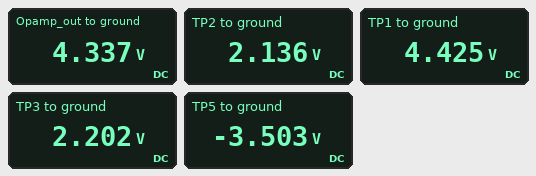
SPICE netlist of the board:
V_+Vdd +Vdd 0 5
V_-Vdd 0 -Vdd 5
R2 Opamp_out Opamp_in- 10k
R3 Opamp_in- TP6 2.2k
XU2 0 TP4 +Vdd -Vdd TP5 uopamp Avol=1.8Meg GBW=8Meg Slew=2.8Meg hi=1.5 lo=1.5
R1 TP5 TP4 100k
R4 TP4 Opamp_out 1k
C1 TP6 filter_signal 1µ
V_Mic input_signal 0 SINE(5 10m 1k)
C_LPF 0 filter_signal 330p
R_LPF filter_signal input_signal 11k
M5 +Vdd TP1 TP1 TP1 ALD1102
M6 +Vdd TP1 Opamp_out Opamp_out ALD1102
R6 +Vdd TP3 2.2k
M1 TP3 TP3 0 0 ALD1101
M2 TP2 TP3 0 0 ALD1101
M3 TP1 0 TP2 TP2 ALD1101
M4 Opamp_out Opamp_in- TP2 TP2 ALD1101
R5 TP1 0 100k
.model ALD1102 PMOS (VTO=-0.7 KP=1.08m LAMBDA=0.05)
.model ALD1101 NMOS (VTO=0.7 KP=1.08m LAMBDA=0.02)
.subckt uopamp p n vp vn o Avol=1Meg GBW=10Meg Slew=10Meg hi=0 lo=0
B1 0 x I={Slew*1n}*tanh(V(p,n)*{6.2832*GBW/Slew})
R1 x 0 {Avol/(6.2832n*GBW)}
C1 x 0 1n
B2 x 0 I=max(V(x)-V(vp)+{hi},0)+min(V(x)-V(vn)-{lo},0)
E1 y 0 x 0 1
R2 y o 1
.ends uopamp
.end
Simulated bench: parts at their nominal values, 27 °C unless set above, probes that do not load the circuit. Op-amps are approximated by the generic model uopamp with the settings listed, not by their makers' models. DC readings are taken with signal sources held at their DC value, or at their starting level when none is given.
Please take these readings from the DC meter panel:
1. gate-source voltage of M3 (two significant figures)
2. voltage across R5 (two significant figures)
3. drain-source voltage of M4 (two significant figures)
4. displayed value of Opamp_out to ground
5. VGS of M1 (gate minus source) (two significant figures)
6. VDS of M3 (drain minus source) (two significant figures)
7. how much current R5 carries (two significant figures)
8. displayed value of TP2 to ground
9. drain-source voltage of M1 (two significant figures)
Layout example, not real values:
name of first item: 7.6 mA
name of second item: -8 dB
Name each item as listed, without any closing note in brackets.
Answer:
gate-source voltage of M3: -2.1 V
voltage across R5: 4.4 V
drain-source voltage of M4: 2.2 V
displayed value of Opamp_out to ground: 4.337 V
VGS of M1 (gate minus source): 2.2 V
VDS of M3 (drain minus source): 2.3 V
how much current R5 carries: 44 µA
displayed value of TP2 to ground: 2.136 V
drain-source voltage of M1: 2.2 V
